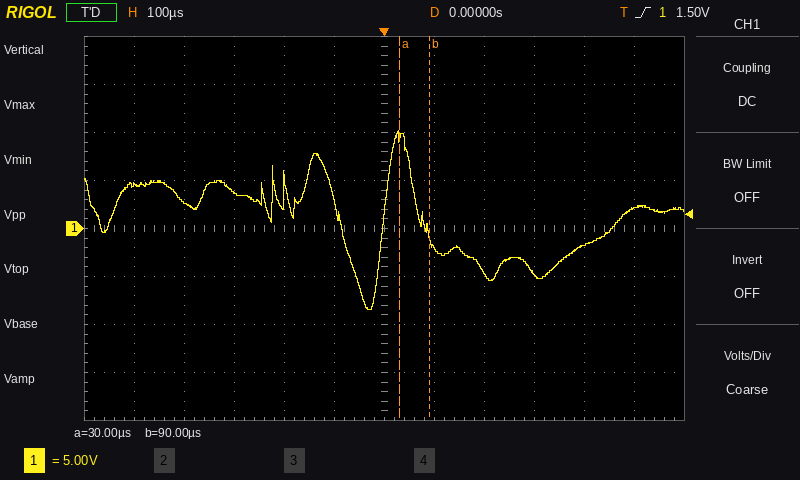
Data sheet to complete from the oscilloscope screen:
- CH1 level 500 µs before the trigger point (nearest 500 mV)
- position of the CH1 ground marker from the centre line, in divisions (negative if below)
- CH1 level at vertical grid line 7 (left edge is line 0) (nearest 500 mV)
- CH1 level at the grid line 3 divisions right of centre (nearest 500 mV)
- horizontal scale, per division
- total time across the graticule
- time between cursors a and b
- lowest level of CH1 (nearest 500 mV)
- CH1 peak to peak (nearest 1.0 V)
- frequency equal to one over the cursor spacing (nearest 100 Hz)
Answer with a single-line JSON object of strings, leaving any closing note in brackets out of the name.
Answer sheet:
{"CH1 level 500 µs before the trigger point": "4.5 V", "position of the CH1 ground marker from the centre line, in divisions": "0.0 div", "CH1 level at vertical grid line 7 (left edge is line 0)": "-2.0 V", "CH1 level at the grid line 3 divisions right of centre": "-5.0 V", "horizontal scale, per division": "100 µs", "total time across the graticule": "1.2 ms", "time between cursors a and b": "60 µs", "lowest level of CH1": "-8.5 V", "CH1 peak to peak": "19.0 V", "frequency equal to one over the cursor spacing": "16.7 kHz"}
